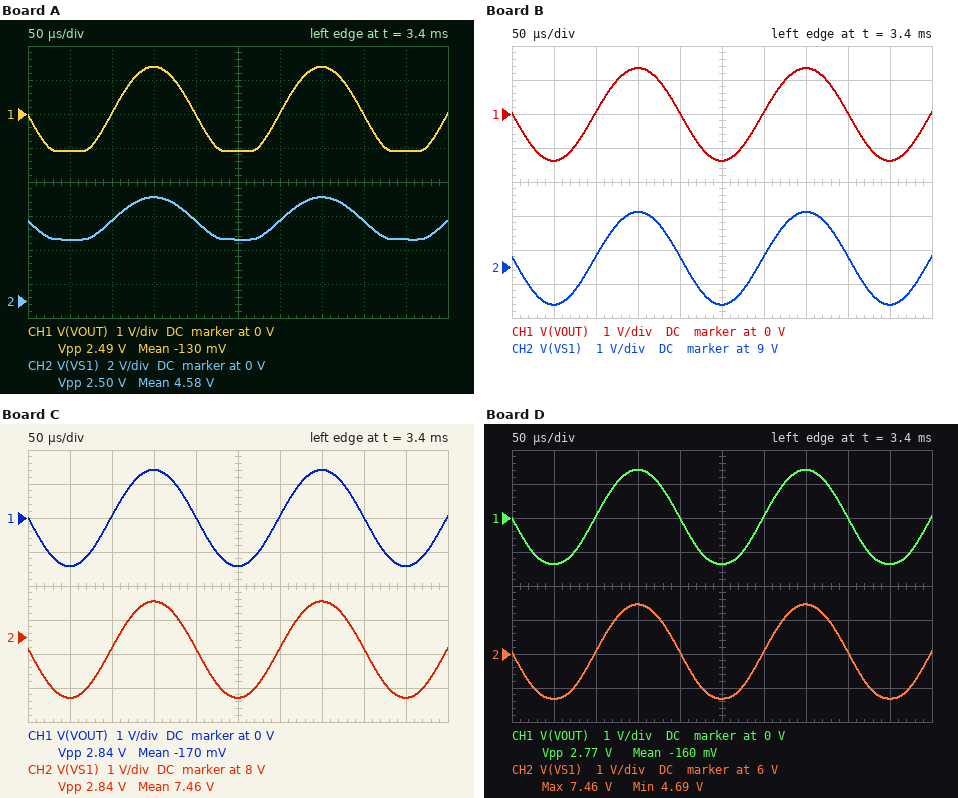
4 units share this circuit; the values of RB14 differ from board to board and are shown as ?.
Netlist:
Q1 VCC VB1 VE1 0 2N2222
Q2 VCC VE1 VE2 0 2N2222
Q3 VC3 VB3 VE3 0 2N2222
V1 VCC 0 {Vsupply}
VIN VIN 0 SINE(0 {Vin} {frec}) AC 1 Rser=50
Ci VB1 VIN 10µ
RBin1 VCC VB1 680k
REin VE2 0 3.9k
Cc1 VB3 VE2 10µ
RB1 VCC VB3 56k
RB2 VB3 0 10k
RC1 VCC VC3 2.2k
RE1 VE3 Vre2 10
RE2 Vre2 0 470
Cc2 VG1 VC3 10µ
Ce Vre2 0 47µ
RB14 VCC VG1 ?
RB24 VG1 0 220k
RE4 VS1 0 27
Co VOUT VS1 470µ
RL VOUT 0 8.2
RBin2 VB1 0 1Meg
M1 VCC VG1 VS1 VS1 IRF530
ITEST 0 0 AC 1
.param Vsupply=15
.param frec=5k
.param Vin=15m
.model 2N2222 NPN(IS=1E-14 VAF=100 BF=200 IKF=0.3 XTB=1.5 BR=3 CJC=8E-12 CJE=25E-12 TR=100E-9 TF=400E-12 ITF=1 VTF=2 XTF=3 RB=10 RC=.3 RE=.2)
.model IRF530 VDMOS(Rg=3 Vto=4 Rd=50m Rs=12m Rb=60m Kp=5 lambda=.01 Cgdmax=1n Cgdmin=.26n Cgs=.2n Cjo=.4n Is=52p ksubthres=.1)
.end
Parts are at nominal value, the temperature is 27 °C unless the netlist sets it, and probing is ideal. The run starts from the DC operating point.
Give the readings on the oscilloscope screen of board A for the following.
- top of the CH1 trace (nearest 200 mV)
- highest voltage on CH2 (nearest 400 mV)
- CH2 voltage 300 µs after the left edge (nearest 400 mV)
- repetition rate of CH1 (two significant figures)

1.4 V
6.0 V
4.8 V
5.0 kHz
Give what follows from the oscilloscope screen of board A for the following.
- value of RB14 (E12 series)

150 kΩ
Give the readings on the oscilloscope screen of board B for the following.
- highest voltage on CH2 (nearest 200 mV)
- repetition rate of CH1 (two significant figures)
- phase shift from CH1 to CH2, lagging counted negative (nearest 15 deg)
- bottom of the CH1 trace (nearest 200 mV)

10.6 V
5.0 kHz
0 deg
-1.4 V
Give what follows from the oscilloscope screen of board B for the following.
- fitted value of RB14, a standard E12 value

22 kΩ
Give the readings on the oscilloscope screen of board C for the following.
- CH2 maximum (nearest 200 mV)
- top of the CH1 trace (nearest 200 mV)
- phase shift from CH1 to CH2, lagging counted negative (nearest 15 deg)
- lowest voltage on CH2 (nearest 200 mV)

9.0 V
1.4 V
0 deg
6.2 V
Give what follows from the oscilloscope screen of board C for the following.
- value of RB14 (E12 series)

56 kΩ
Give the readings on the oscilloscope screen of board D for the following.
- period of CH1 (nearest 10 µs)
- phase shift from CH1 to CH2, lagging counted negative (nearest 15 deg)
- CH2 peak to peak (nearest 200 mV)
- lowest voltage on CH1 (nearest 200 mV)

200 µs
0 deg
2.8 V
-1.4 V
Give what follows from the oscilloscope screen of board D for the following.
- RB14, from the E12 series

100 kΩ
